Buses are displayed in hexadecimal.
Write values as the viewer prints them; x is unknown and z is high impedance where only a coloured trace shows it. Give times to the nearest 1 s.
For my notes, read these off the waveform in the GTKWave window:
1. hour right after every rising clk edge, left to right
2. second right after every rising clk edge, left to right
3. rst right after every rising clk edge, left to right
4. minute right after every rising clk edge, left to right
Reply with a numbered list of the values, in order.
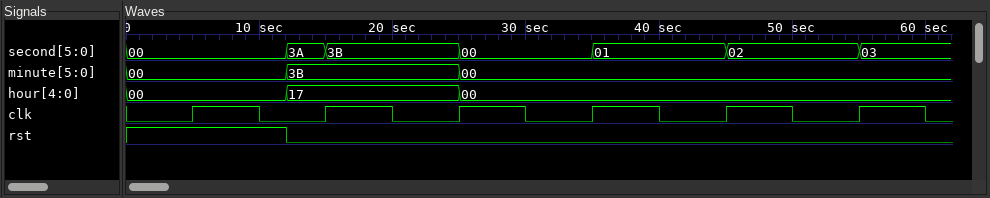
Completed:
1. 00, 17, 00, 00, 00, 00
2. 00, 3B, 00, 01, 02, 03
3. 1 0 0 0 0 0
4. 00, 3B, 00, 00, 00, 00
